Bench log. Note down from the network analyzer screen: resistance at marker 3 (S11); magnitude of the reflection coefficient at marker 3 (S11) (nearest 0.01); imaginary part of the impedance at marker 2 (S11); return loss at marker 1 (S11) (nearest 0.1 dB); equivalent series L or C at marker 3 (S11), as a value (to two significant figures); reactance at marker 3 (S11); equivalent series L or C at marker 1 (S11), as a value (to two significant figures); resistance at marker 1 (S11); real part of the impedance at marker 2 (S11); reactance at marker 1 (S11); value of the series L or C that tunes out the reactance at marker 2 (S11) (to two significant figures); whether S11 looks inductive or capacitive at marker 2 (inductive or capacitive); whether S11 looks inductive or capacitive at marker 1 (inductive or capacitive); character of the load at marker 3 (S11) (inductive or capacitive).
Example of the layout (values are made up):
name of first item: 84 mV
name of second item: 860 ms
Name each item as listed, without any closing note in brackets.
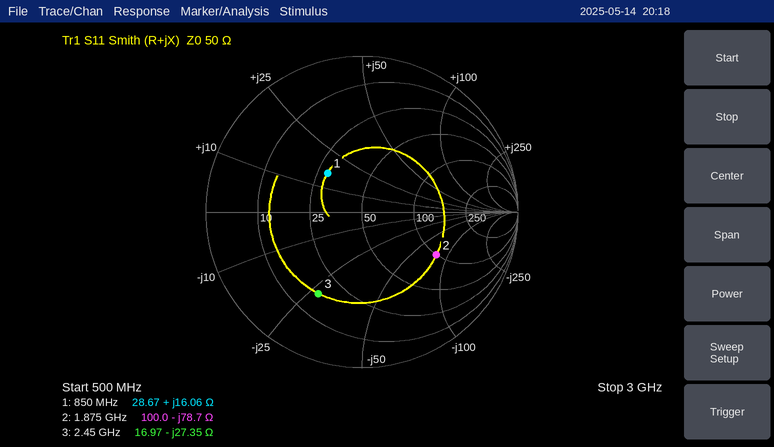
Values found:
resistance at marker 3: 16.97 Ω
magnitude of the reflection coefficient at marker 3 (S11): 0.59
imaginary part of the impedance at marker 2: -78.7 Ω
return loss at marker 1 (S11): 9.6 dB
equivalent series L or C at marker 3 (S11), as a value: 2.4 pF
reactance at marker 3: -27.35 Ω
equivalent series L or C at marker 1 (S11), as a value: 3.0 nH
resistance at marker 1: 28.67 Ω
real part of the impedance at marker 2: 100.0 Ω
reactance at marker 1: +16.06 Ω
value of the series L or C that tunes out the reactance at marker 2 (S11): 6.7 nH
whether S11 looks inductive or capacitive at marker 2: capacitive
whether S11 looks inductive or capacitive at marker 1: inductive
character of the load at marker 3 (S11): capacitive
